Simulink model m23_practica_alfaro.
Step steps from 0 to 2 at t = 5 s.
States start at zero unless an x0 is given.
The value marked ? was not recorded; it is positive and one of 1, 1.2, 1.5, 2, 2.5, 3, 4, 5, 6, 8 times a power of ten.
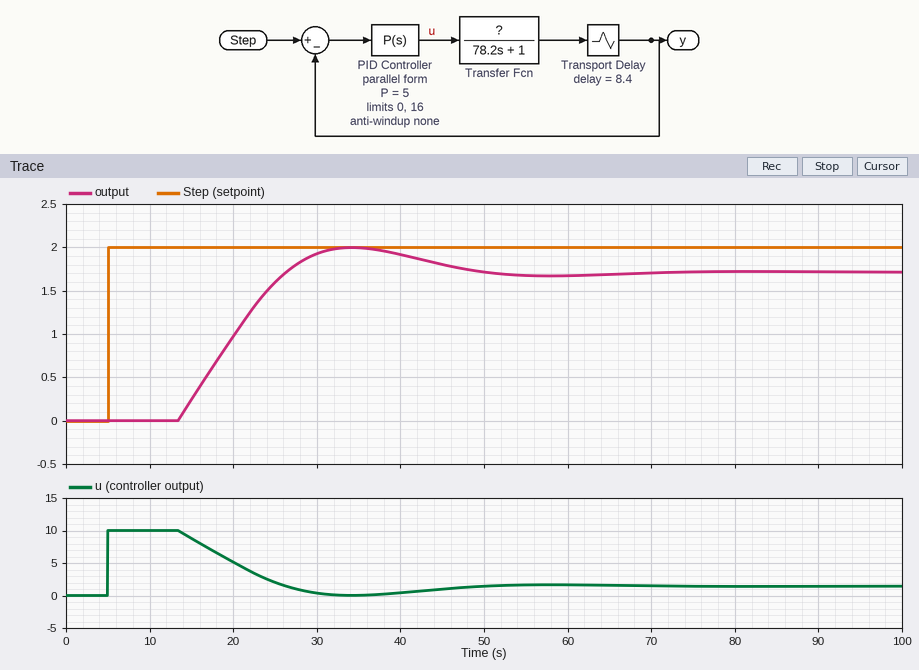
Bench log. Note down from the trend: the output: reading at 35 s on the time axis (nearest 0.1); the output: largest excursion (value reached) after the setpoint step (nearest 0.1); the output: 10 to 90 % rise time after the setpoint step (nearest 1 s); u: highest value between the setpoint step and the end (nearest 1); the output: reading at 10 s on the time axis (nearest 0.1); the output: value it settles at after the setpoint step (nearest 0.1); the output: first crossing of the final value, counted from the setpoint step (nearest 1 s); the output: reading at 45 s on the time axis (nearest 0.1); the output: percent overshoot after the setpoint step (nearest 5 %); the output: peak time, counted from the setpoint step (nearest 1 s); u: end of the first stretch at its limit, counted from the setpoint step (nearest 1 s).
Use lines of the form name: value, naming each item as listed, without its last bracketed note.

the output: reading at 35 s on the time axis: 2.0
the output: largest excursion (value reached) after the setpoint step: 2.0
the output: 10 to 90 % rise time after the setpoint step: 10 s
u: highest value between the setpoint step and the end: 10
the output: reading at 10 s on the time axis: 0.0
the output: value it settles at after the setpoint step: 1.7
the output: first crossing of the final value, counted from the setpoint step: 21 s
the output: reading at 45 s on the time axis: 1.8
the output: percent overshoot after the setpoint step: 15 %
the output: peak time, counted from the setpoint step: 29 s
u: end of the first stretch at its limit, counted from the setpoint step: 9 s
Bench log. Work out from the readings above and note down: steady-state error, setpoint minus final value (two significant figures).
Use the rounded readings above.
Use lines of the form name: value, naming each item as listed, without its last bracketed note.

steady-state error, setpoint minus final value: 0.30
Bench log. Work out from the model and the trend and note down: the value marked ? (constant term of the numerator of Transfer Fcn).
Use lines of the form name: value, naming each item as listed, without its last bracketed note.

the value marked ?: 1.2
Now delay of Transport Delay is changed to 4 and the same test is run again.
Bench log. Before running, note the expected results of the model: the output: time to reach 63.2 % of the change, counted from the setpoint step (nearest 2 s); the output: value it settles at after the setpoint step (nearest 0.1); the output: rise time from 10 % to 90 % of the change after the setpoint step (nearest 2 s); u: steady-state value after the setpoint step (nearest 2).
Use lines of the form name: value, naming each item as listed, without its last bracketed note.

the output: time to reach 63.2 % of the change, counted from the setpoint step: 12 s
the output: value it settles at after the setpoint step: 1.7
the output: rise time from 10 % to 90 % of the change after the setpoint step: 16 s
u: steady-state value after the setpoint step: 2
